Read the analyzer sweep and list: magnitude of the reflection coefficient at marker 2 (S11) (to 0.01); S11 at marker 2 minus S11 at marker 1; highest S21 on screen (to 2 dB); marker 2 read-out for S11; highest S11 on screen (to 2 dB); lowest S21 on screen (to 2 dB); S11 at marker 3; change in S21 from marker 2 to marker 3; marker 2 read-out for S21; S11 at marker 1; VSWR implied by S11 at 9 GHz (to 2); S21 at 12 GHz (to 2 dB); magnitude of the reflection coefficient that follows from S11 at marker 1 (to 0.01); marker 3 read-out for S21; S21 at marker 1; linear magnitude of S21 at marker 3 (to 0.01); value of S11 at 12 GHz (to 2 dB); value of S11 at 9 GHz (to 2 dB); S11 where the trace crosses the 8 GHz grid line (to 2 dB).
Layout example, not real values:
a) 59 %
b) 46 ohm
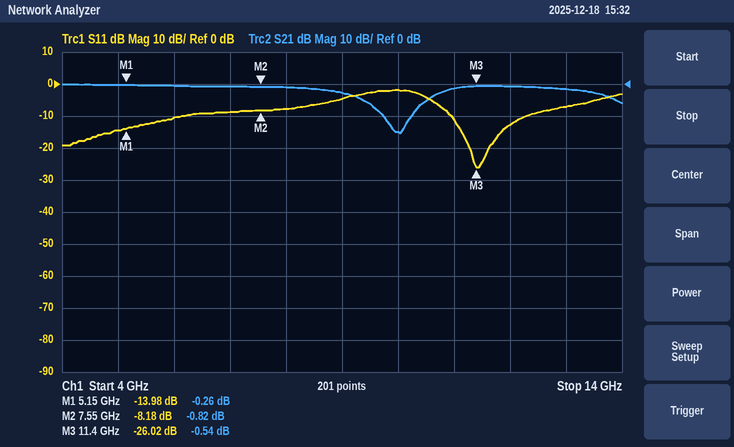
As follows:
a) 0.39
b) 5.80 dB
c) 0 dB
d) -8.18 dB
e) -2 dB
f) -16 dB
g) -26.02 dB
h) 0.28 dB
i) -0.82 dB
j) -13.98 dB
k) 4
l) 0 dB
m) 0.20
n) -0.54 dB
o) -0.26 dB
p) 0.94
q) -12 dB
r) -4 dB
s) -8 dB
